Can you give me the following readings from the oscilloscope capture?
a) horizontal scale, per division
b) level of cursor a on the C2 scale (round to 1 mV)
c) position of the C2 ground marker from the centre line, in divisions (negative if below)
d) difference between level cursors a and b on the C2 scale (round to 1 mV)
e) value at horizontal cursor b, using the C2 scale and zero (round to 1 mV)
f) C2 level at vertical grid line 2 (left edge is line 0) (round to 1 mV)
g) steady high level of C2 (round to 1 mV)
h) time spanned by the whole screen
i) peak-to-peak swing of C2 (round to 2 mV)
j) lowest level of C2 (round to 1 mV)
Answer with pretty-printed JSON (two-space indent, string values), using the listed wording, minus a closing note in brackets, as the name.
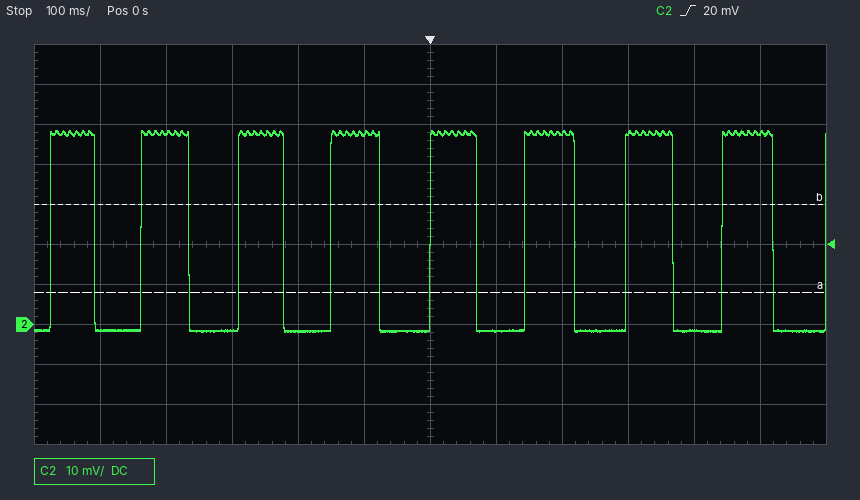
{
  "horizontal scale, per division": "100 ms",
  "level of cursor a on the C2 scale": "8 mV",
  "position of the C2 ground marker from the centre line, in divisions": "-2.0 div",
  "difference between level cursors a and b on the C2 scale": "22 mV",
  "value at horizontal cursor b, using the C2 scale and zero": "30 mV",
  "C2 level at vertical grid line 2 (left edge is line 0)": "48 mV",
  "steady high level of C2": "48 mV",
  "time spanned by the whole screen": "1.2 s",
  "peak-to-peak swing of C2": "50 mV",
  "lowest level of C2": "-2 mV"
}
